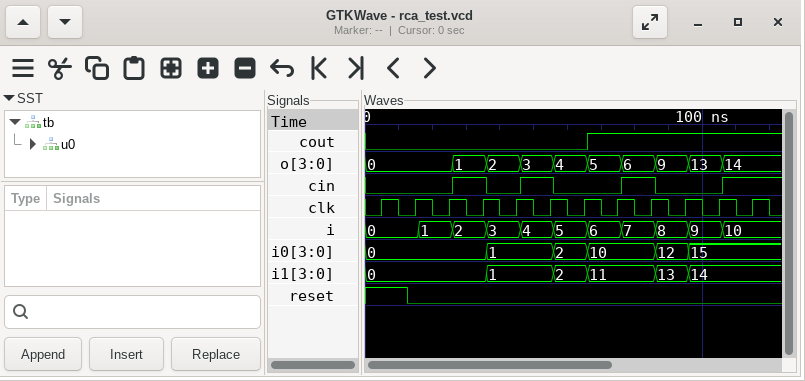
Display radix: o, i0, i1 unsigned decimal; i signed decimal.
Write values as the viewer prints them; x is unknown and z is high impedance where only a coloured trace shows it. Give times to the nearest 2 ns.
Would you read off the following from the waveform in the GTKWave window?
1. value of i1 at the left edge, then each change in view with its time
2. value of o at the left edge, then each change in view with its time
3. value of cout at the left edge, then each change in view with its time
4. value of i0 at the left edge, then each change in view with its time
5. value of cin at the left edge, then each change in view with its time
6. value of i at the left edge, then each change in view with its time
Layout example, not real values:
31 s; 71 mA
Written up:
0, 1 at 36 ns, 2 at 56 ns, 11 at 66 ns, 13 at 86 ns, 14 at 96 ns; 0, 1 at 26 ns, 2 at 36 ns, 3 at 46 ns, 4 at 56 ns, 5 at 66 ns, 6 at 76 ns, 9 at 86 ns, 13 at 96 ns, 14 at 106 ns; 0, 1 at 66 ns; 0, 1 at 36 ns, 2 at 56 ns, 10 at 66 ns, 12 at 86 ns, 15 at 96 ns; 0, 1 at 26 ns, 0 at 36 ns, 1 at 46 ns, 0 at 56 ns, 1 at 76 ns, 0 at 86 ns, 1 at 106 ns; 0, 1 at 16 ns, 2 at 26 ns, 3 at 36 ns, 4 at 46 ns, 5 at 56 ns, 6 at 66 ns, 7 at 76 ns, 8 at 86 ns, 9 at 96 ns, 10 at 106 ns
